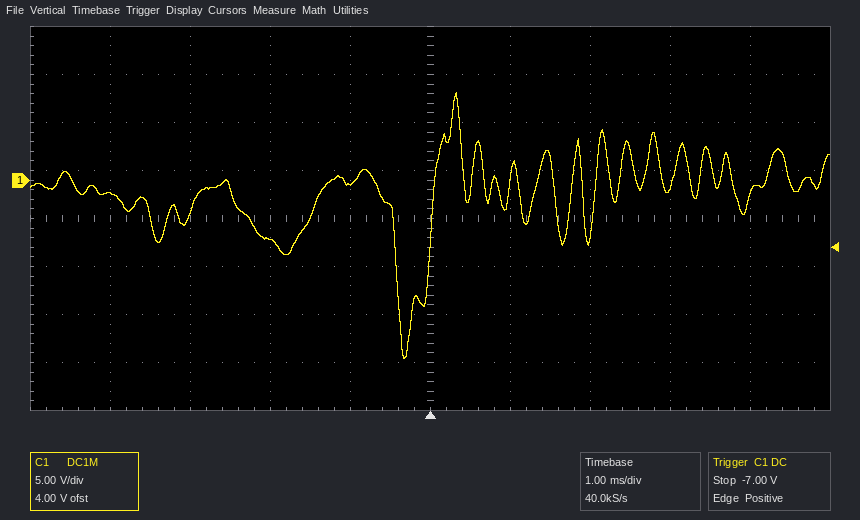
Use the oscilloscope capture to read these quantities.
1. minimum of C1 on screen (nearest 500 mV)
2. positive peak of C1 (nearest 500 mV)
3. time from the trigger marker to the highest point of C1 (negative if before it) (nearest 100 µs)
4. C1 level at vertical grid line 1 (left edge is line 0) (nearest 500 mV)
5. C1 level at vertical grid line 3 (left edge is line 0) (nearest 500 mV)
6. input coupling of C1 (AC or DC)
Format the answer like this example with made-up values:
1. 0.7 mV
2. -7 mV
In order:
1. -18.5 V
2. 9.0 V
3. +300 µs
4. -1.5 V
5. -6.0 V
6. DC
